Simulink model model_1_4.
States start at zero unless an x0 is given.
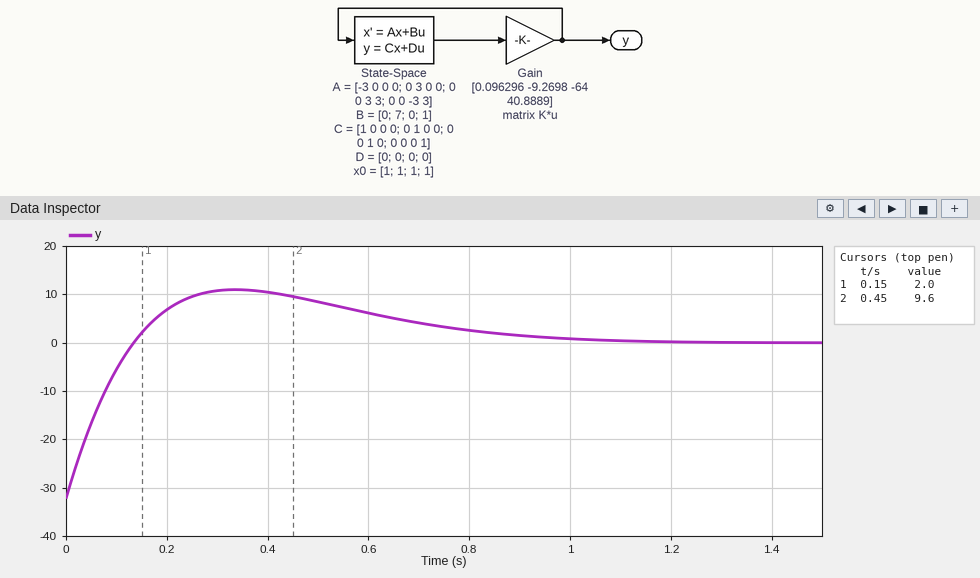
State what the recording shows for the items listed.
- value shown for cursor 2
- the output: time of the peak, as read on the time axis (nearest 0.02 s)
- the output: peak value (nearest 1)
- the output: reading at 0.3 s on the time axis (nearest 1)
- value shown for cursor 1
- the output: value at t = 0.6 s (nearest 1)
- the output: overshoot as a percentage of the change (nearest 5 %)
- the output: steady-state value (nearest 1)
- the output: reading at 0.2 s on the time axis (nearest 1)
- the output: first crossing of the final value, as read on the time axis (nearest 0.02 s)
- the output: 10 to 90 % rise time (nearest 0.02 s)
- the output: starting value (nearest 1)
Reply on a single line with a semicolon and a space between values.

9.6; 0.34 s; 11; 11; 2.0; 6; 35 %; 0; 7; 0.14 s; 0.10 s; -32
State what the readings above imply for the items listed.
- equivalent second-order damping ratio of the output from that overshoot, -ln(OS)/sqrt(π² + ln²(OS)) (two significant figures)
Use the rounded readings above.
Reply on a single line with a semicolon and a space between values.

0.32
